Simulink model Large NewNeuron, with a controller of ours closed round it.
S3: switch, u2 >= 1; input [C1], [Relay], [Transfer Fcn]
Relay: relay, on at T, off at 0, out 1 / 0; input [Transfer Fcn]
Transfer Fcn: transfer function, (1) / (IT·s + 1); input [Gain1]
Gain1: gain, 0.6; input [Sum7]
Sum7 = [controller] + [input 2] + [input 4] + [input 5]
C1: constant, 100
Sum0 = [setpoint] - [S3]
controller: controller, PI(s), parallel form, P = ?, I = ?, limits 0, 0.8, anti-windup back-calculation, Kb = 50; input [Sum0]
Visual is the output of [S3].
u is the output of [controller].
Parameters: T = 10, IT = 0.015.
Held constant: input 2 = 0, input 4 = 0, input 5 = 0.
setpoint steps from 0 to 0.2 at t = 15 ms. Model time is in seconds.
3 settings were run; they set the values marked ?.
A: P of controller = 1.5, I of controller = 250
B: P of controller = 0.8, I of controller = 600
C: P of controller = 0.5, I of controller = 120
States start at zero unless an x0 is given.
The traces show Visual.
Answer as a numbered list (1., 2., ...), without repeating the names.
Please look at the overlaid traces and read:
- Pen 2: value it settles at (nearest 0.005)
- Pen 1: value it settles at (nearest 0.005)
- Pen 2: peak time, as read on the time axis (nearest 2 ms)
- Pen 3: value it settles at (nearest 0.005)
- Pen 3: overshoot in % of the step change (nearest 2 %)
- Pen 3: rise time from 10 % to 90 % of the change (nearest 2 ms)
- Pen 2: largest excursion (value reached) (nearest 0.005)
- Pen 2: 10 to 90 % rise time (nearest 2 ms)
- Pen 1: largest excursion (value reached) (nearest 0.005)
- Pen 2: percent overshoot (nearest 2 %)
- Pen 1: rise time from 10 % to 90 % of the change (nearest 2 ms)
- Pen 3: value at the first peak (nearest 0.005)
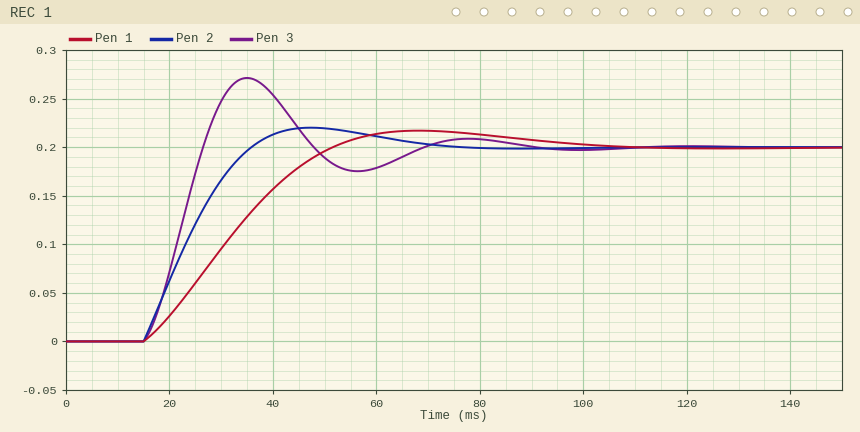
1. 0.200
2. 0.200
3. 48 ms
4. 0.200
5. 36 %
6. 8 ms
7. 0.220
8. 16 ms
9. 0.215
10. 10 %
11. 26 ms
12. 0.270
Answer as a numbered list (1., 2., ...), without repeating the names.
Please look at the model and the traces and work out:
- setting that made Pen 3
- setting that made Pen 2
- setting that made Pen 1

1. B
2. A
3. C
